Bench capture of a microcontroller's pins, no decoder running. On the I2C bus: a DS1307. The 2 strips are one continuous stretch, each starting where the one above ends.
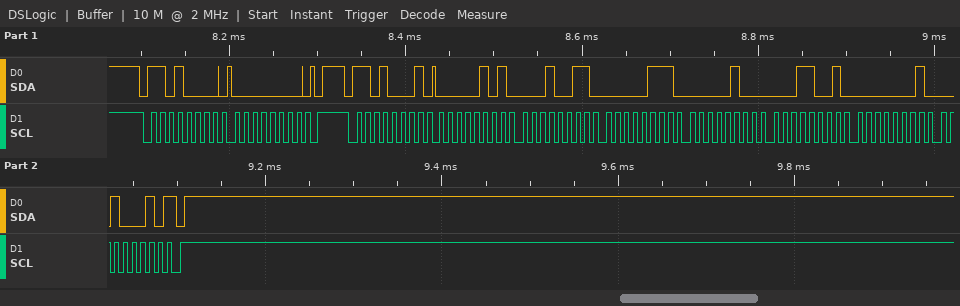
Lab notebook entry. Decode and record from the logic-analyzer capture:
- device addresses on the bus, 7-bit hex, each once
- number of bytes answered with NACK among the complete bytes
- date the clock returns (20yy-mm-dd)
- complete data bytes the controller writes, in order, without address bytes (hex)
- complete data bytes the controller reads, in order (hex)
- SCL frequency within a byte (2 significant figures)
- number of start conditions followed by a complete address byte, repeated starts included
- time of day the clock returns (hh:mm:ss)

0x68
1
2022-01-19
00
05 13 07 04 19 01 22
100 kHz
2
07:13:05
